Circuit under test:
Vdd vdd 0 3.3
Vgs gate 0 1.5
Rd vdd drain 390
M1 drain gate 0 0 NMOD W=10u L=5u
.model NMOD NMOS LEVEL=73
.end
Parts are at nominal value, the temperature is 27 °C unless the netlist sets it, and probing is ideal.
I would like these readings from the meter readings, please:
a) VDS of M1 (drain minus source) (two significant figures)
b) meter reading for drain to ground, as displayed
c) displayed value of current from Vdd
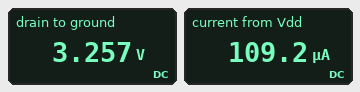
3.3 V
3.257 V
109.2 µA
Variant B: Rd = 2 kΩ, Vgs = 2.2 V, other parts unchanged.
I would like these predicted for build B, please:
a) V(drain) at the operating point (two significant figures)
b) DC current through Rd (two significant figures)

2.7 V
320 µA
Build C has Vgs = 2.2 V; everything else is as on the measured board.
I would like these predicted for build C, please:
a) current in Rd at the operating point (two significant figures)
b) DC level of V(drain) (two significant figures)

320 µA
3.2 V
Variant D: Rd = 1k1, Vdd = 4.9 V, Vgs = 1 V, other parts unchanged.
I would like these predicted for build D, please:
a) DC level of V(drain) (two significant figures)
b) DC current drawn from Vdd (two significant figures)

4.9 V
24 µA
